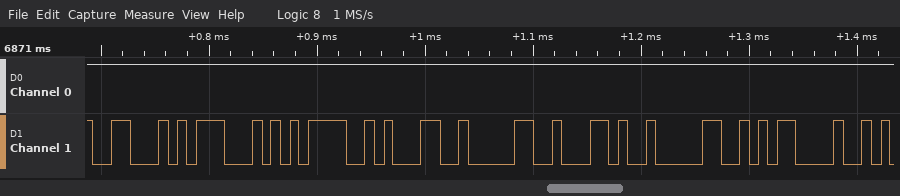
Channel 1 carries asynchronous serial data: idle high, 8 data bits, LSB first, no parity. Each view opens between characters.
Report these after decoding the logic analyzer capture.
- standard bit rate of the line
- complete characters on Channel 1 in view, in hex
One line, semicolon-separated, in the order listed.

115200 baud; 46, 47, 3D, 31, 30, 2C, 30, 0D
